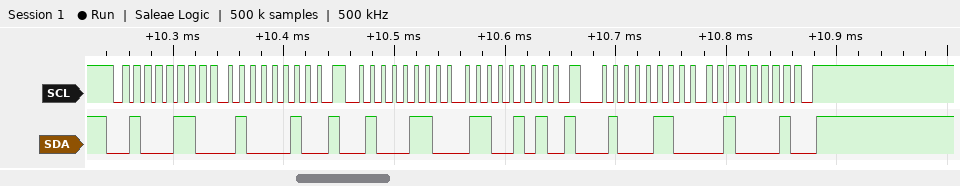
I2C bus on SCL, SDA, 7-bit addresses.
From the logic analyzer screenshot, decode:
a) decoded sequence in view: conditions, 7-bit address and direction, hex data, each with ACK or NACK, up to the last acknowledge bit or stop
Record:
start, address 23 write ACK, 42 ACK, repeated start, address 23 write ACK, 65 ACK, repeated start, address 23 write ACK, 21 ACK, stop
